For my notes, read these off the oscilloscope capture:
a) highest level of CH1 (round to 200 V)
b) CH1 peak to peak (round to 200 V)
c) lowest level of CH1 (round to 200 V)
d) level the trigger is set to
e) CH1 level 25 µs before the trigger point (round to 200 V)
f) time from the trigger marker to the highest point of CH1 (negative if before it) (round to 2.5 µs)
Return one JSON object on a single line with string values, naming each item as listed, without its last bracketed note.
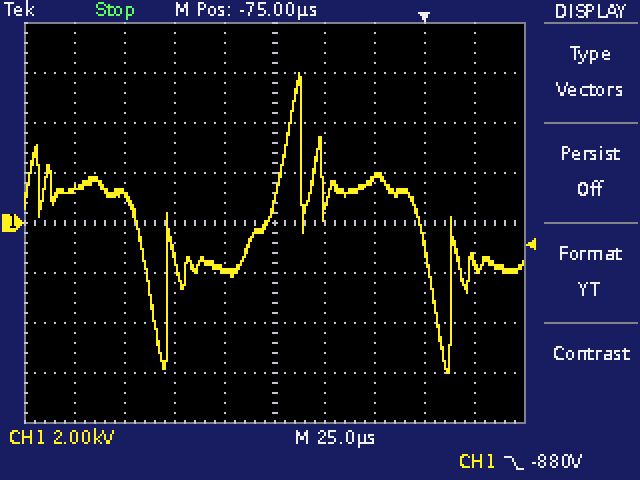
{"highest level of CH1": "6.0 kV", "CH1 peak to peak": "12.0 kV", "lowest level of CH1": "-6.0 kV", "level the trigger is set to": "-880 V", "CH1 level 25 µs before the trigger point": "1.8 kV", "time from the trigger marker to the highest point of CH1 (negative if before it)": "-62.5 µs"}
